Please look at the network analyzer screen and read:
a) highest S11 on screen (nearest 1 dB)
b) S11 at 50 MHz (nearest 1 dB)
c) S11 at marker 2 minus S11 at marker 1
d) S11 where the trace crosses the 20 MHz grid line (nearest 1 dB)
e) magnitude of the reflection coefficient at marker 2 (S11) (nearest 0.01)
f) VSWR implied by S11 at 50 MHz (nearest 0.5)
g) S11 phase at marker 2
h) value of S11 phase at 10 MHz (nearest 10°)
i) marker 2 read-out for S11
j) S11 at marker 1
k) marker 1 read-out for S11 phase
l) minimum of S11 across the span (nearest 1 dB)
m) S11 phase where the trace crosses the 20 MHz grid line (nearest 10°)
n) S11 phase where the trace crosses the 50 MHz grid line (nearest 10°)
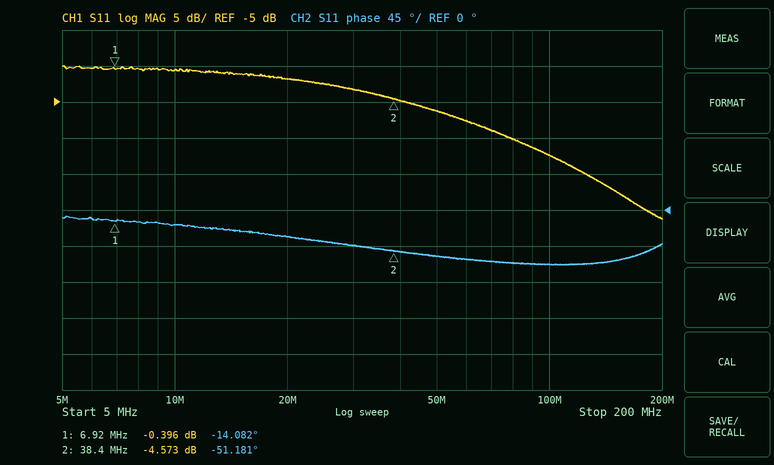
0 dB
-6 dB
-4.177 dB
-2 dB
0.59
3.0
-51.181°
-20°
-4.573 dB
-0.396 dB
-14.082°
-21 dB
-30°
-60°
